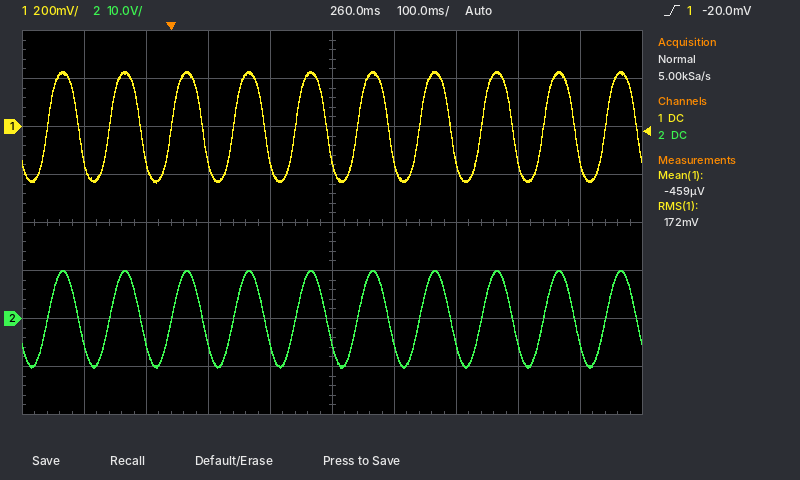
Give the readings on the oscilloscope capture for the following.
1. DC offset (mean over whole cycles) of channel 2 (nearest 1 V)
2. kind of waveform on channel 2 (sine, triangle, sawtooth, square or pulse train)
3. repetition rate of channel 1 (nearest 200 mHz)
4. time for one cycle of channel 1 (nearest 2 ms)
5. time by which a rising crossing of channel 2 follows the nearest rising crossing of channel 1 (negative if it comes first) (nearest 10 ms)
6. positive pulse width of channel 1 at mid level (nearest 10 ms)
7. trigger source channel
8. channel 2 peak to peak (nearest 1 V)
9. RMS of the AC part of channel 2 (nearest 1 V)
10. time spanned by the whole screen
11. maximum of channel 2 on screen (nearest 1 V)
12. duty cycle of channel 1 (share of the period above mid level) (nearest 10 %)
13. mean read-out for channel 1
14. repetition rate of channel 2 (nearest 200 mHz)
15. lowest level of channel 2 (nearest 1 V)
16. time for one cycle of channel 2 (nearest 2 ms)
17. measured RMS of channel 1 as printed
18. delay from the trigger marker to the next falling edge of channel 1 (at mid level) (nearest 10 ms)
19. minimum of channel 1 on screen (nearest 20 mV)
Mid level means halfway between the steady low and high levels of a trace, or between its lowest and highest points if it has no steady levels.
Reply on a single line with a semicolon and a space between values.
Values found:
0 V; sine; 10.0 Hz; 100 ms; 0 ms; 50 ms; channel 1; 20 V; 7 V; 1 s; 10 V; 50 %; -459 µV; 10.0 Hz; -10 V; 100 ms; 172 mV; 50 ms; -240 mV
